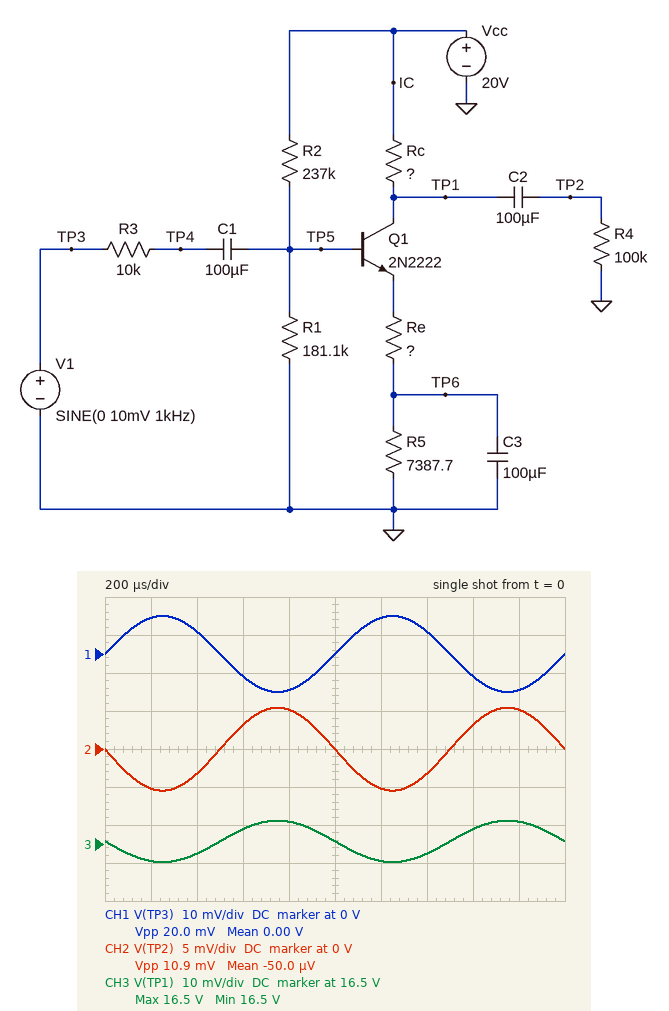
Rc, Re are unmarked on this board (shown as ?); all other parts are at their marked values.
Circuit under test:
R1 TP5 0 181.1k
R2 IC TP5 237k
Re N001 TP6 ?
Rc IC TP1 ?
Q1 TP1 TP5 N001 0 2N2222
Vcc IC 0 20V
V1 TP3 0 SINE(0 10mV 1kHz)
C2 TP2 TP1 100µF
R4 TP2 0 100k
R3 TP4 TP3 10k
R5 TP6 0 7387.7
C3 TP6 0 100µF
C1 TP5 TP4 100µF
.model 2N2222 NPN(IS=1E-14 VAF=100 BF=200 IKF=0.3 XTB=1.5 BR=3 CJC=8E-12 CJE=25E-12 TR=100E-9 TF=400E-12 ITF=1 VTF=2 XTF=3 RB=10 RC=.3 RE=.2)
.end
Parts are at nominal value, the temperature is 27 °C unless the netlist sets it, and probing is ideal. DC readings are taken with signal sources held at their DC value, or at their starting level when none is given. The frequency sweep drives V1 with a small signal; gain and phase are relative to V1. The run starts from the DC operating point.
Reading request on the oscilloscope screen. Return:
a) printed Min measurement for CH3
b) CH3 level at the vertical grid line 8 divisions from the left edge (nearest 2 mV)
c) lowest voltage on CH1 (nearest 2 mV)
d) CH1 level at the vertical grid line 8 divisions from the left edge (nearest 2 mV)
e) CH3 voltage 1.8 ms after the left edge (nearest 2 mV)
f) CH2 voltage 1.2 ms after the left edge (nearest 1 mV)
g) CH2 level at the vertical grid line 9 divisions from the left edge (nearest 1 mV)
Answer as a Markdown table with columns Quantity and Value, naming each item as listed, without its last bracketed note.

| Quantity | Value |
|---|---|
| printed Min measurement for CH3 | 16.5 V |
| CH3 level at the vertical grid line 8 divisions from the left edge | 16.504 V |
| lowest voltage on CH1 | -10 mV |
| CH1 level at the vertical grid line 8 divisions from the left edge | -6 mV |
| CH3 voltage 1.8 ms after the left edge | 16.506 V |
| CH2 voltage 1.2 ms after the left edge | -5 mV |
| CH2 level at the vertical grid line 9 divisions from the left edge | 5 mV |
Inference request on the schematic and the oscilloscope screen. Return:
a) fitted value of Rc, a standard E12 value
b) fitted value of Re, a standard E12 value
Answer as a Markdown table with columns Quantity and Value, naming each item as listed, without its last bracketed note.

| Quantity | Value |
|---|---|
| fitted value of Rc, a standard E12 value | 10 kΩ |
| fitted value of Re, a standard E12 value | 15 kΩ |
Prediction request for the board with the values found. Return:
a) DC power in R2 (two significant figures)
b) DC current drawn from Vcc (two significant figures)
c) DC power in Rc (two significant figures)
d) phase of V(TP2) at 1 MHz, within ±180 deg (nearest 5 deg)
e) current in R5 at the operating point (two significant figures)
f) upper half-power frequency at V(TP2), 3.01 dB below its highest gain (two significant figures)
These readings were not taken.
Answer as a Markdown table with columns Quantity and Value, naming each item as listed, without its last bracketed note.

| Quantity | Value |
|---|---|
| DC power in R2 | 560 µW |
| DC current drawn from Vcc | 400 µA |
| DC power in Rc | 1.2 mW |
| phase of V(TP2) at 1 MHz, within ±180 deg | 130 deg |
| current in R5 at the operating point | 350 µA |
| upper half-power frequency at V(TP2), 3.01 dB below its highest gain | 5.2 MHz |
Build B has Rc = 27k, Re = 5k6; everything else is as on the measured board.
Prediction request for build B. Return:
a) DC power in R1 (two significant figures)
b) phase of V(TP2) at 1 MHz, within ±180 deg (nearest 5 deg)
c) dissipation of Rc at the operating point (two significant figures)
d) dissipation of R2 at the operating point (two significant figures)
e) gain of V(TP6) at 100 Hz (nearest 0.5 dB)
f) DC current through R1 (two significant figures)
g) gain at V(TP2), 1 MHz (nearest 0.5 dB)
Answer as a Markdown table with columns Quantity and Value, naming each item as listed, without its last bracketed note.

| Quantity | Value |
|---|---|
| DC power in R1 | 290 µW |
| phase of V(TP2) at 1 MHz, within ±180 deg | 10 deg |
| dissipation of Rc at the operating point | 6.6 mW |
| dissipation of R2 at the operating point | 690 µW |
| gain of V(TP6) at 100 Hz | -61.0 dB |
| DC current through R1 | 40 µA |
| gain at V(TP2), 1 MHz | -11.0 dB |
